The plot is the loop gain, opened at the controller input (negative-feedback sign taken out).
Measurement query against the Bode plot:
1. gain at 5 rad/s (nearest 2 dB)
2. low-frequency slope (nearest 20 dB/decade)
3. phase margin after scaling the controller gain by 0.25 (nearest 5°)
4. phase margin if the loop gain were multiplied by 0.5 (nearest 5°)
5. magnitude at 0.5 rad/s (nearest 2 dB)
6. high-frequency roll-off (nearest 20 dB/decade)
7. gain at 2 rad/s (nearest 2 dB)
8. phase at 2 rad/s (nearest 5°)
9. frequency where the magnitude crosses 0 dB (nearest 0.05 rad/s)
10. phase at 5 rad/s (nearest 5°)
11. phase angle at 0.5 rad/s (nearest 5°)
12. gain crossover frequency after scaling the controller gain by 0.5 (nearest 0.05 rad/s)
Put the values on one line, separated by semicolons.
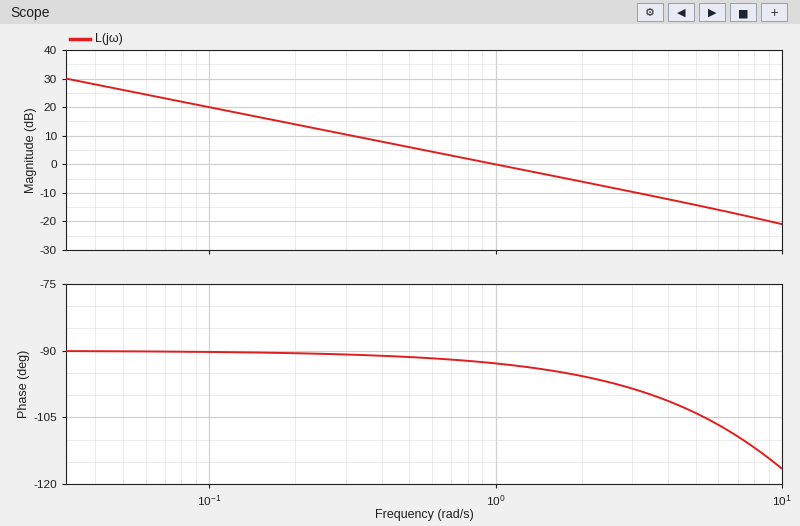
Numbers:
-14 dB; -20 dB/decade; 90°; 90°; 6 dB; -20 dB/decade; -6 dB; -95°; 1.00 rad/s; -105°; -90°; 0.50 rad/s
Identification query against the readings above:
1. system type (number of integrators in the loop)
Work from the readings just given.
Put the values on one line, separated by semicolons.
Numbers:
1
